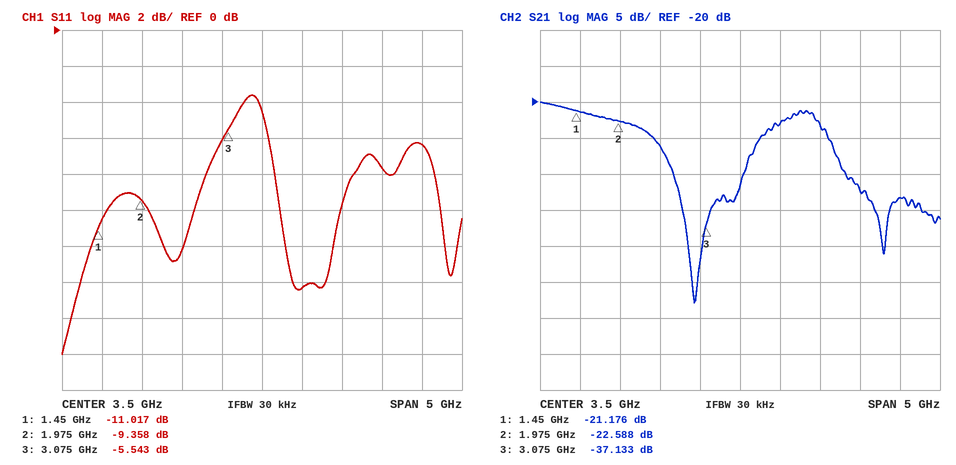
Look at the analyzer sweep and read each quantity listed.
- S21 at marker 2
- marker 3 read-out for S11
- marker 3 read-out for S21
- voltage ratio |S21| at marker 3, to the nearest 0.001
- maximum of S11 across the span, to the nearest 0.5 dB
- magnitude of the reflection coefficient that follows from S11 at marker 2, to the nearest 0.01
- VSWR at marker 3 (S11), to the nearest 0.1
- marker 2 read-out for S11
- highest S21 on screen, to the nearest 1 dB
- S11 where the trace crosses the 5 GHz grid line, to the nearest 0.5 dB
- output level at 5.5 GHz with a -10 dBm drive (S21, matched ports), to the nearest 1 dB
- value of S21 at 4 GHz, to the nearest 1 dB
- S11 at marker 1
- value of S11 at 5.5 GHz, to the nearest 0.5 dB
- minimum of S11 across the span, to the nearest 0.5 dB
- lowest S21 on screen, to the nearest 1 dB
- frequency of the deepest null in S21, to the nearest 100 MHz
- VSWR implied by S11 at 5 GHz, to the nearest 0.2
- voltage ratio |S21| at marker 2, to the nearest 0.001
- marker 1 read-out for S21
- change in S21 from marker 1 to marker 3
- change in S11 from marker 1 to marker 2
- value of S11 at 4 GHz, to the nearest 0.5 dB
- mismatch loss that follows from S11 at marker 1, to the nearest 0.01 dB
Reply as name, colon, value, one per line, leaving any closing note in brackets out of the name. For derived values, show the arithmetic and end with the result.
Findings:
S21 at marker 2: -22.588 dB
marker 3 read-out for S11: -5.543 dB
marker 3 read-out for S21: -37.133 dB
voltage ratio |S21| at marker 3, to the nearest 0.001: 10^(-37.133/20) ≈ 0.014
maximum of S11 across the span, to the nearest 0.5 dB: -3.5 dB
magnitude of the reflection coefficient that follows from S11 at marker 2, to the nearest 0.01: 10^(-9.358/20) ≈ 0.34
VSWR at marker 3 (S11), to the nearest 0.1: (1 + 0.5283)/(1 − 0.5283) ≈ 3.2
marker 2 read-out for S11: -9.358 dB
highest S21 on screen, to the nearest 1 dB: -20 dB
S11 where the trace crosses the 5 GHz grid line, to the nearest 0.5 dB: -7.5 dB
output level at 5.5 GHz with a -10 dBm drive (S21, matched ports), to the nearest 1 dB: -10 dBm + (-33 dB) = -43 dBm
value of S21 at 4 GHz, to the nearest 1 dB: -23 dB
S11 at marker 1: -11.017 dB
value of S11 at 5.5 GHz, to the nearest 0.5 dB: -6.5 dB
minimum of S11 across the span, to the nearest 0.5 dB: -18.0 dB
lowest S21 on screen, to the nearest 1 dB: -48 dB
frequency of the deepest null in S21, to the nearest 100 MHz: 2.9 GHz
VSWR implied by S11 at 5 GHz, to the nearest 0.2: |Γ| = 10^(-7.5/20) = 0.4217; VSWR = (1 + 0.4217)/(1 − 0.4217) ≈ 2.46, so 2.4 to the nearest 0.2
voltage ratio |S21| at marker 2, to the nearest 0.001: 10^(-22.588/20) ≈ 0.074
marker 1 read-out for S21: -21.176 dB
change in S21 from marker 1 to marker 3: -37.133 − (-21.176) = -15.957 dB
change in S11 from marker 1 to marker 2: -9.358 − (-11.017) = 1.659 dB
value of S11 at 4 GHz, to the nearest 0.5 dB: -14.5 dB
mismatch loss that follows from S11 at marker 1, to the nearest 0.01 dB: −10 log10(1 − 10^(-11.017/10)) ≈ 0.36 dB
